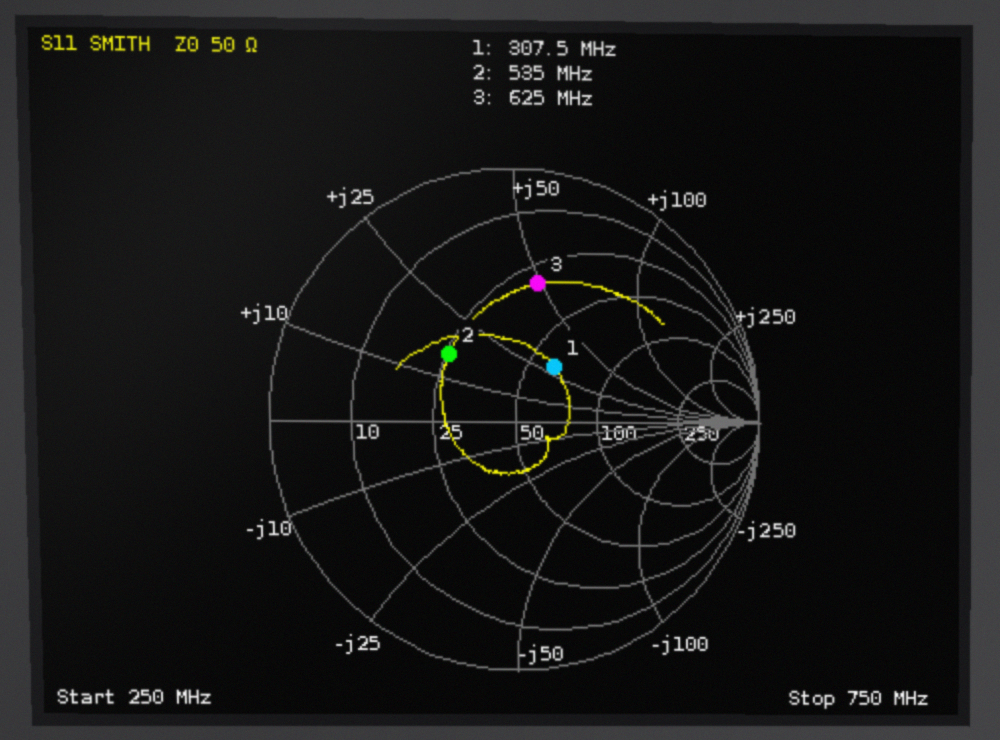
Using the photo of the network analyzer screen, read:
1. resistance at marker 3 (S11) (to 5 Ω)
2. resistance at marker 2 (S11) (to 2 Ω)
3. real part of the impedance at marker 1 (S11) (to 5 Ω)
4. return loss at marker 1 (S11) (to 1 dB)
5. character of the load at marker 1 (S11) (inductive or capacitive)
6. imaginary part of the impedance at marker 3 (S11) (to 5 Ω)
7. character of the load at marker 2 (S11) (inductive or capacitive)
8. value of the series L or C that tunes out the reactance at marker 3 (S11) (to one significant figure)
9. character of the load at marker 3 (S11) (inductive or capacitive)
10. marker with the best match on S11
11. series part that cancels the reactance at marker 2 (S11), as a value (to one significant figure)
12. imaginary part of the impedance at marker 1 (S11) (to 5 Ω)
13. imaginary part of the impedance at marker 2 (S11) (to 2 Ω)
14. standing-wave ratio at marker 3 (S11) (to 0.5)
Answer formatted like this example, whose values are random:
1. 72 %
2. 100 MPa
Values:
1. 30 Ω
2. 26 Ω
3. 60 Ω
4. 11 dB
5. inductive
6. +50 Ω
7. inductive
8. 5 pF
9. inductive
10. marker 1
11. 20 pF
12. +30 Ω
13. +16 Ω
14. 3.5
